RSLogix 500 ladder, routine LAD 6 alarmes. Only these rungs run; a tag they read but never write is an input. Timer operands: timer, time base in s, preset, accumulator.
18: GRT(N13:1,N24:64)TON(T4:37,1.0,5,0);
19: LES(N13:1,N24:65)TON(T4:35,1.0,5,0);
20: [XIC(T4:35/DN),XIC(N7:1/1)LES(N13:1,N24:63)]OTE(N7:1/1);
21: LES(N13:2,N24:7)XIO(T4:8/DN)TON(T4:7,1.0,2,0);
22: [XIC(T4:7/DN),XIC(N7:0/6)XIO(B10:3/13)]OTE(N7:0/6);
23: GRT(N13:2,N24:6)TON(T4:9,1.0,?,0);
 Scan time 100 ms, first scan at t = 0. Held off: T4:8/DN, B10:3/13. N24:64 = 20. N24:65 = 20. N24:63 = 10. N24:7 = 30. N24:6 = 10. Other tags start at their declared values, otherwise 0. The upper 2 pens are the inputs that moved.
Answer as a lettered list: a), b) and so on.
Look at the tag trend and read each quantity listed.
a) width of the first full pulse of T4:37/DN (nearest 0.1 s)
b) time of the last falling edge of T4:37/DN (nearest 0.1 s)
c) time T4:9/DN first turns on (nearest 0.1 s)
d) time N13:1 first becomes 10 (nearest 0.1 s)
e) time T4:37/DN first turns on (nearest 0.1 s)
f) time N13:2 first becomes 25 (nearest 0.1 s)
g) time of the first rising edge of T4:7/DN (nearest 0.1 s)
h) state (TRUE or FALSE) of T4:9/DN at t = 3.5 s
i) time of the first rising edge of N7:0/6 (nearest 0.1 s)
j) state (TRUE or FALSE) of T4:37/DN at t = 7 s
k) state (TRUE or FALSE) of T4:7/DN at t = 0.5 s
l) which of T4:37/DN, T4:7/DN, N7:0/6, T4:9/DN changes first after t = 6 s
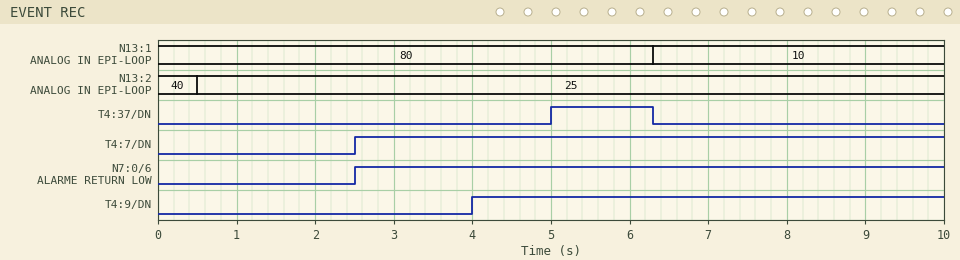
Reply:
a) 1.3 s
b) 6.3 s
c) 4.0 s
d) 6.3 s
e) 5.0 s
f) 0.5 s
g) 2.5 s
h) FALSE
i) 2.5 s
j) FALSE
k) FALSE
l) T4:37/DN
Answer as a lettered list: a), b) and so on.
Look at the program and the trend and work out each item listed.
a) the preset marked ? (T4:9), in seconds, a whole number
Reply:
a) 4 s
